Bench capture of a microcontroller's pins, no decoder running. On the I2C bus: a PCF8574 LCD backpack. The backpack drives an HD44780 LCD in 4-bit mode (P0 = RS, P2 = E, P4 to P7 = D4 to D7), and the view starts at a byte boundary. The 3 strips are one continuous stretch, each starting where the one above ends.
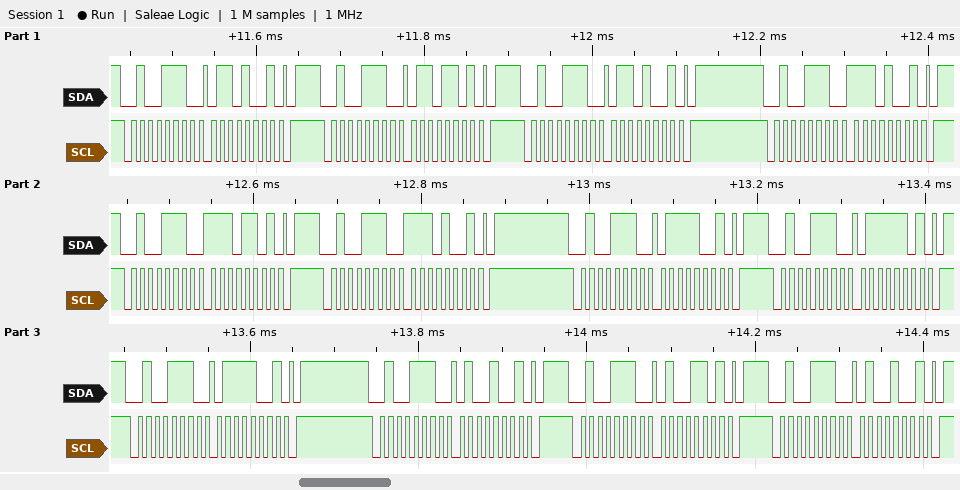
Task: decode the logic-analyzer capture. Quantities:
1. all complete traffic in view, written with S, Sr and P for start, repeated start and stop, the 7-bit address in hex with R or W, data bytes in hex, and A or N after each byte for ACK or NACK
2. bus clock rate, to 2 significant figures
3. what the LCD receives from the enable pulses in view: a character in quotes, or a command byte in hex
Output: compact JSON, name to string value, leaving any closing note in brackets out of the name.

{"all complete traffic in view, written with S, Sr and P for start, repeated start and stop, the 7-bit address in hex with R or W, data bytes in hex, and A or N after each byte for ACK or NACK": "S 27W A 69 A P S 27W A 6D A P S 27W A 69 A P S 27W A E9 A P S 27W A ED A P S 27W A E9 A P S 27W A 79 A P S 27W A 7D A P S 27W A 79 A P S 27W A 49 A P S 27W A 4D A P S 27W A 49 A P", "bus clock rate, to 2 significant figures": "100 kHz", "what the LCD receives from the enable pulses in view: a character in quotes, or a command byte in hex": "'n' 't'"}
